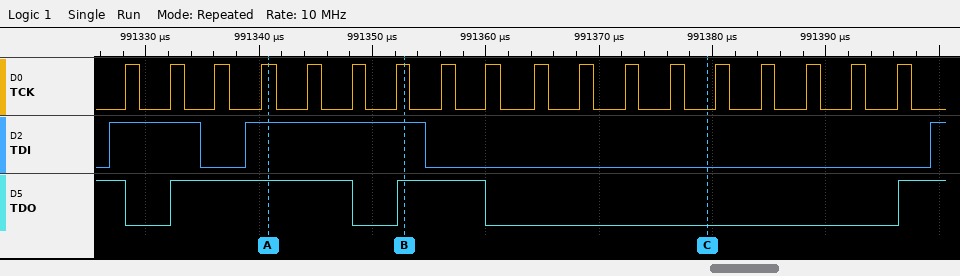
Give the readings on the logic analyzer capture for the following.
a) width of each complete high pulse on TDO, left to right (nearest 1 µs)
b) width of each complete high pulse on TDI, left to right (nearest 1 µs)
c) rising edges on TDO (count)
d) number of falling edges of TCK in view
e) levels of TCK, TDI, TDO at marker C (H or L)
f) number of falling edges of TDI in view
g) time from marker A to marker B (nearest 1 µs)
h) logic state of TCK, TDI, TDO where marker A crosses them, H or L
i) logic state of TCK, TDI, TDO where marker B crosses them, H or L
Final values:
16 µs, 8 µs
8 µs, 16 µs
3
18
TCK=L, TDI=L, TDO=L
2
12 µs
TCK=H, TDI=H, TDO=H
TCK=H, TDI=H, TDO=H
